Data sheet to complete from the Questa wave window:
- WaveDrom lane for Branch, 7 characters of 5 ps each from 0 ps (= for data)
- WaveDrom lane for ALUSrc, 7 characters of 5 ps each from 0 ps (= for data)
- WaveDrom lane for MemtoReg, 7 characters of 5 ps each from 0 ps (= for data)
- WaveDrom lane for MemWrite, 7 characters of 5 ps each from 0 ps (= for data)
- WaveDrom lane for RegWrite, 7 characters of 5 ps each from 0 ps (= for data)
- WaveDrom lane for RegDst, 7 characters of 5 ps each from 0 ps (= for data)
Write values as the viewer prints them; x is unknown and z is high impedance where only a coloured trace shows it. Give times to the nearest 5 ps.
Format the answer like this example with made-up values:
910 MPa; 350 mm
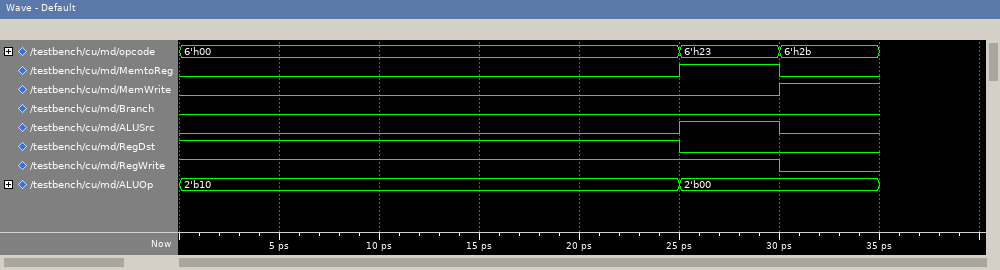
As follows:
{name: 'Branch', wave: '0......'}; {name: 'ALUSrc', wave: '0....10'}; {name: 'MemtoReg', wave: '0....10'}; {name: 'MemWrite', wave: '0.....1'}; {name: 'RegWrite', wave: '1.....0'}; {name: 'RegDst', wave: '1....0.'}
